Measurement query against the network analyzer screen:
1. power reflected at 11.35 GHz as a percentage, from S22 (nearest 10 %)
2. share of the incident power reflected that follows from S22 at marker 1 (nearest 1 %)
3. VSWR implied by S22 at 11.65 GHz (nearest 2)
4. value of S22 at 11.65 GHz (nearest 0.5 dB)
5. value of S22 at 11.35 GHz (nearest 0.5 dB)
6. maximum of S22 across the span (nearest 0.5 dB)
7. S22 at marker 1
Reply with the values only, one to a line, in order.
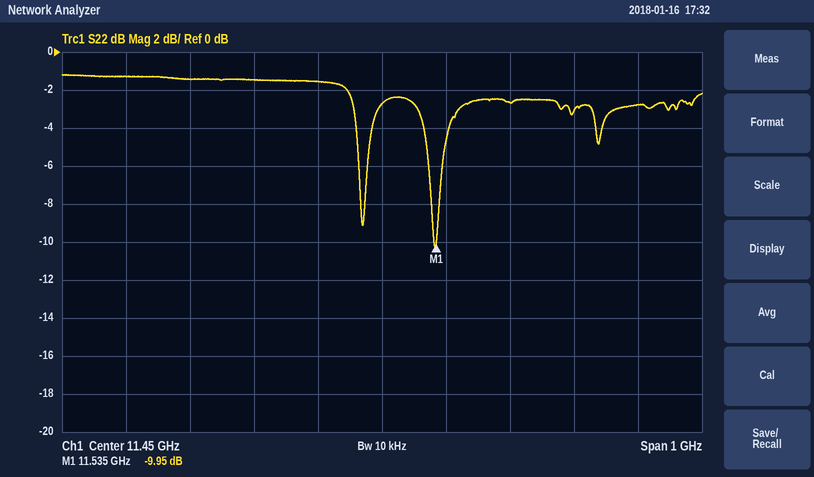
70 %
10 %
6
-2.5 dB
-1.5 dB
-1.0 dB
-9.95 dB
